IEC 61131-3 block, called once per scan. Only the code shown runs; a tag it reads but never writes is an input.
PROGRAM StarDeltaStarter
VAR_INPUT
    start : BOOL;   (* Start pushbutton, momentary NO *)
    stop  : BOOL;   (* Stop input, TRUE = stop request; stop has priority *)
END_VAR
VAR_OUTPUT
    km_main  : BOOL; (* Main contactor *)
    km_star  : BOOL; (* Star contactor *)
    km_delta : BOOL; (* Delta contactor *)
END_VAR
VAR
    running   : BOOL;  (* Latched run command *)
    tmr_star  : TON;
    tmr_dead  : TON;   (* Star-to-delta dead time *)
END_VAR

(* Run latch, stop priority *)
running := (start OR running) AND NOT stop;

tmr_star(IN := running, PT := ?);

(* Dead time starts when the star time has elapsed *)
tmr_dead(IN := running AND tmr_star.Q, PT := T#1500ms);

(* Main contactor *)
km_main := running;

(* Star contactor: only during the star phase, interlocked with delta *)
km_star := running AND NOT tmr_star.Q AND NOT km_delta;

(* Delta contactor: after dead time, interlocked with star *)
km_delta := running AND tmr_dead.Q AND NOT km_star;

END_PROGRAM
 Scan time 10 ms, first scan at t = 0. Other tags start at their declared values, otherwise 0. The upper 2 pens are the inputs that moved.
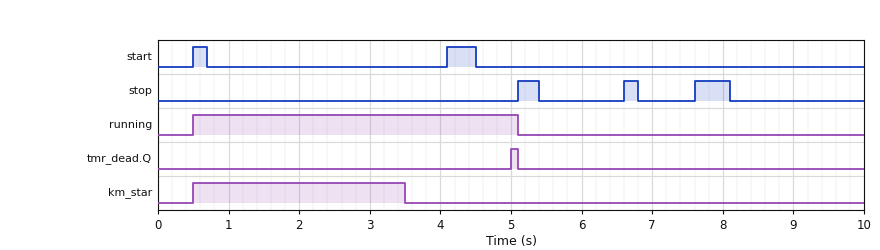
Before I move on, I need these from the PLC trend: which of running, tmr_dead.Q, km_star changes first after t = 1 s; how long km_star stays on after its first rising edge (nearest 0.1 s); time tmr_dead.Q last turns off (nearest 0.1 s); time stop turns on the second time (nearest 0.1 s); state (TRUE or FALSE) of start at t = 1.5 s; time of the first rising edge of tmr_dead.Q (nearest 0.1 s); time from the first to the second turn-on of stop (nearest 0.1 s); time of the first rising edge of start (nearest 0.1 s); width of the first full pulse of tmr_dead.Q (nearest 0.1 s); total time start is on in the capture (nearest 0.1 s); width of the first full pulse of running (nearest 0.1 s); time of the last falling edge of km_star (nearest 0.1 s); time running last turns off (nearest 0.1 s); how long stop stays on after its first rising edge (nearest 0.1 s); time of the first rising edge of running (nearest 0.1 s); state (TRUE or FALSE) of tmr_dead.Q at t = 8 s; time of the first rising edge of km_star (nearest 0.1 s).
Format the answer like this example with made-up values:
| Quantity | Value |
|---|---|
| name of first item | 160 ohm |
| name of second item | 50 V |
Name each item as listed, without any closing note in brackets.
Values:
| Quantity | Value |
|---|---|
| which of running, tmr_dead.Q, km_star changes first after t = 1 s | km_star |
| how long km_star stays on after its first rising edge | 3.0 s |
| time tmr_dead.Q last turns off | 5.1 s |
| time stop turns on the second time | 6.6 s |
| state (TRUE or FALSE) of start at t = 1.5 s | FALSE |
| time of the first rising edge of tmr_dead.Q | 5.0 s |
| time from the first to the second turn-on of stop | 1.5 s |
| time of the first rising edge of start | 0.5 s |
| width of the first full pulse of tmr_dead.Q | 0.1 s |
| total time start is on in the capture | 0.6 s |
| width of the first full pulse of running | 4.6 s |
| time of the last falling edge of km_star | 3.5 s |
| time running last turns off | 5.1 s |
| how long stop stays on after its first rising edge | 0.3 s |
| time of the first rising edge of running | 0.5 s |
| state (TRUE or FALSE) of tmr_dead.Q at t = 8 s | FALSE |
| time of the first rising edge of km_star | 0.5 s |
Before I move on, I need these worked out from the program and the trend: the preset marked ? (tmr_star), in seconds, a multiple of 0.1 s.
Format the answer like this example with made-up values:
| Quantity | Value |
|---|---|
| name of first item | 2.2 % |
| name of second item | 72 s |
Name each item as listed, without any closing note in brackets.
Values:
| Quantity | Value |
|---|---|
| the preset marked ? (tmr_star), in seconds, a multiple of 0.1 s | 3.0 s |
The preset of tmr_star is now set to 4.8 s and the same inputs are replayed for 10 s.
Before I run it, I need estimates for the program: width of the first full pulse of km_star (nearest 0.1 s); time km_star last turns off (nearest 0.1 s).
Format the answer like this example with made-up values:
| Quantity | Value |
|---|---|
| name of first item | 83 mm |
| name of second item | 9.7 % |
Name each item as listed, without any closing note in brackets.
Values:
| Quantity | Value |
|---|---|
| width of the first full pulse of km_star | 4.6 s |
| time km_star last turns off | 5.1 s |
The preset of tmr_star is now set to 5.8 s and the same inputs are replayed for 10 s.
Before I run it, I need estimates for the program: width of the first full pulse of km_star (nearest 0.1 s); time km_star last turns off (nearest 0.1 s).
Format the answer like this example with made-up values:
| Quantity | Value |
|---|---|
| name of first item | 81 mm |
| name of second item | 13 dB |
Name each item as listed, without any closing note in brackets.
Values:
| Quantity | Value |
|---|---|
| width of the first full pulse of km_star | 4.6 s |
| time km_star last turns off | 5.1 s |
